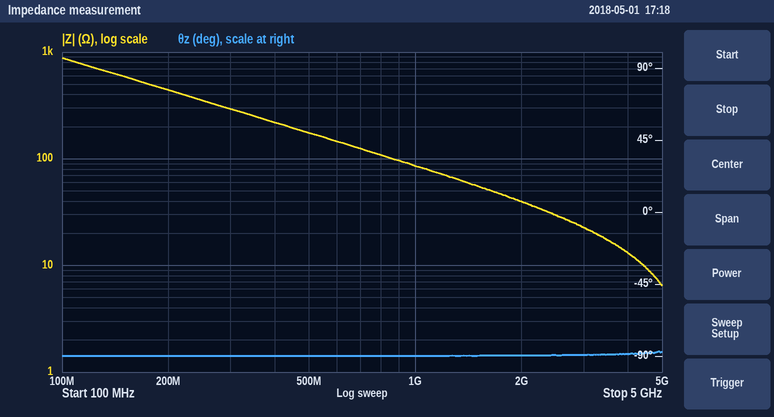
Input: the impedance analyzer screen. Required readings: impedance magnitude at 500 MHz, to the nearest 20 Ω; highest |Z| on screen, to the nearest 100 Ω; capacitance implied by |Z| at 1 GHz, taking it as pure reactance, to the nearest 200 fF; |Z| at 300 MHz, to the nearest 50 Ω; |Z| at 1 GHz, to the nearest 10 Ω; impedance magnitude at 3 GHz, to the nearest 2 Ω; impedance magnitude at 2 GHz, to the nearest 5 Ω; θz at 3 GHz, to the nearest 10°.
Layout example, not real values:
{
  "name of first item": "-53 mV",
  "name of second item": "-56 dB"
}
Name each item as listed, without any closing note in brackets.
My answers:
{
  "impedance magnitude at 500 MHz, to the nearest 20 Ω": "180 Ω",
  "highest |Z| on screen, to the nearest 100 Ω": "900 Ω",
  "capacitance implied by |Z| at 1 GHz, taking it as pure reactance, to the nearest 200 fF": "1.8 pF",
  "|Z| at 300 MHz, to the nearest 50 Ω": "300 Ω",
  "|Z| at 1 GHz, to the nearest 10 Ω": "90 Ω",
  "impedance magnitude at 3 GHz, to the nearest 2 Ω": "22 Ω",
  "impedance magnitude at 2 GHz, to the nearest 5 Ω": "40 Ω",
  "θz at 3 GHz, to the nearest 10°": "-90°"
}
